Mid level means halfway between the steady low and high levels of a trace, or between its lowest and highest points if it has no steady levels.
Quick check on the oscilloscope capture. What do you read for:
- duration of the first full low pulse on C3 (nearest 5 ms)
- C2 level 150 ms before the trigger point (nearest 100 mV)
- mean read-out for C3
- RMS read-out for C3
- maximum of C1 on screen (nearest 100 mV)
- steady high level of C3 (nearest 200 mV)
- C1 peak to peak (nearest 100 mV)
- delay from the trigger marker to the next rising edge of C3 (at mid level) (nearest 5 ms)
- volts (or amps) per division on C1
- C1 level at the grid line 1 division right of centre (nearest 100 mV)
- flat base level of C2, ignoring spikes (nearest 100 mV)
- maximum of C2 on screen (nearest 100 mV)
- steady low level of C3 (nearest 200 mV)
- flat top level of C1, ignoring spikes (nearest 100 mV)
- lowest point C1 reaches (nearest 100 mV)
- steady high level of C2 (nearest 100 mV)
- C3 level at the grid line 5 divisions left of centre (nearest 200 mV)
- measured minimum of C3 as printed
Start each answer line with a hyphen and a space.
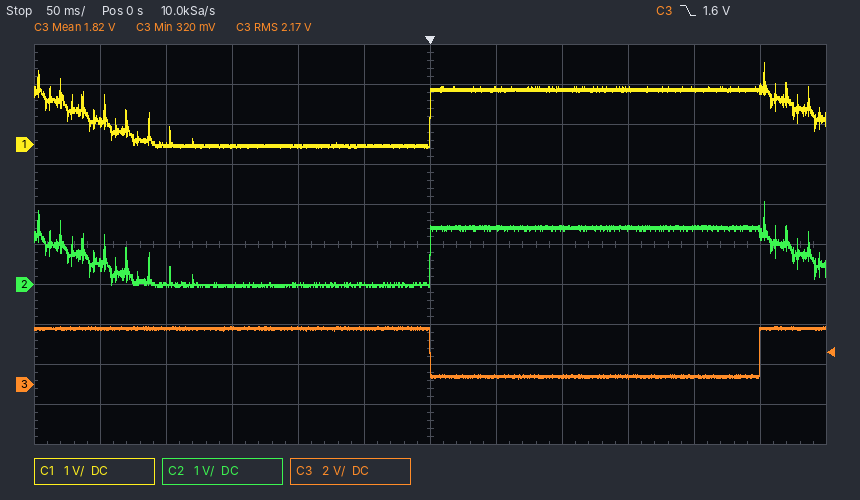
- 250 ms
- 0.0 V
- 1.82 V
- 2.17 V
- 2.0 V
- 2.8 V
- 2.1 V
- 250 ms
- 1 V
- 1.4 V
- 0.0 V
- 2.1 V
- 400 mV
- 1.4 V
- -100 mV
- 1.4 V
- 2.8 V
- 320 mV
